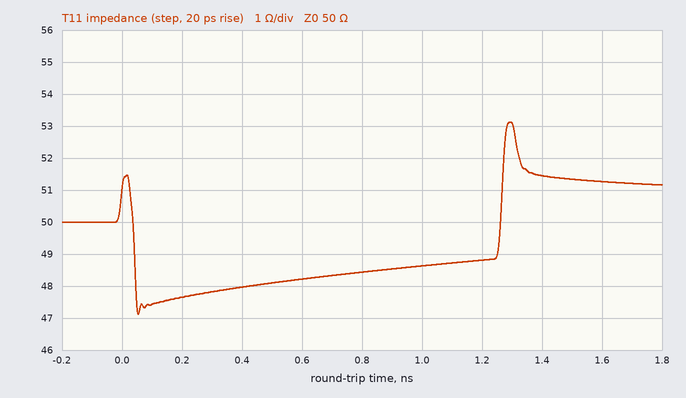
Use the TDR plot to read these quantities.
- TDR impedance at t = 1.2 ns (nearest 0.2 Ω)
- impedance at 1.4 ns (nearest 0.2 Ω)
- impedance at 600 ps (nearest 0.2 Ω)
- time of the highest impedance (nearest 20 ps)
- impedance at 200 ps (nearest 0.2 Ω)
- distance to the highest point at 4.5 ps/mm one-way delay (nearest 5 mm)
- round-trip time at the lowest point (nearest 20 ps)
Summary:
48.8 Ω
51.4 Ω
48.2 Ω
1.30 ns
47.6 Ω
145 mm
60 ps
